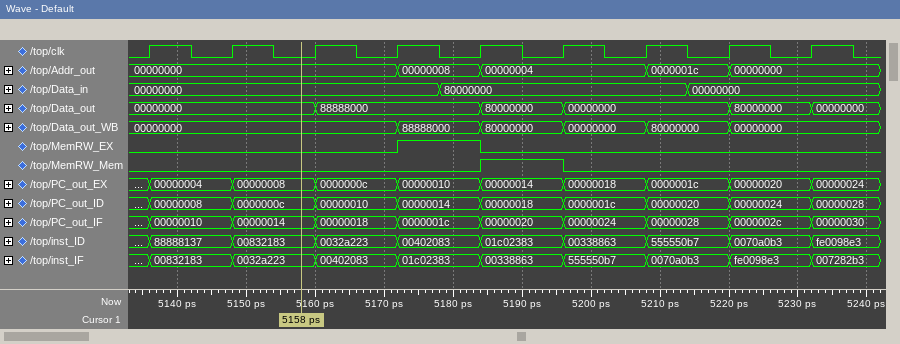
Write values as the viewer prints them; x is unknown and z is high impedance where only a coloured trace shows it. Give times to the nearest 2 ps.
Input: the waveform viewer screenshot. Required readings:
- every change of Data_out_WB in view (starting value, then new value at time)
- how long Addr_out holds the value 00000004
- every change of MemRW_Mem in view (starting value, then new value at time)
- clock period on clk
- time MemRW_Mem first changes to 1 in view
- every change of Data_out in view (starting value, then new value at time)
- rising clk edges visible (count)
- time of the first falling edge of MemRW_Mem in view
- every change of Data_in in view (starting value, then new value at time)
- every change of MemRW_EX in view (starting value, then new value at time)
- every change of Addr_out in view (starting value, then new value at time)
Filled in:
00000000, 88888000 at 5172 ps, 80000000 at 5184 ps, 00000000 at 5196 ps, 80000000 at 5208 ps, 00000000 at 5220 ps
24 ps
0, 1 at 5184 ps, 0 at 5196 ps
12 ps
5184 ps
00000000, 88888000 at 5160 ps, 80000000 at 5184 ps, 00000000 at 5196 ps, 80000000 at 5220 ps, 00000000 at 5232 ps
9
5196 ps
00000000, 80000000 at 5178 ps, 00000000 at 5214 ps
0, 1 at 5172 ps, 0 at 5184 ps
00000000, 00000008 at 5172 ps, 00000004 at 5184 ps, 0000001c at 5208 ps, 00000000 at 5220 ps
